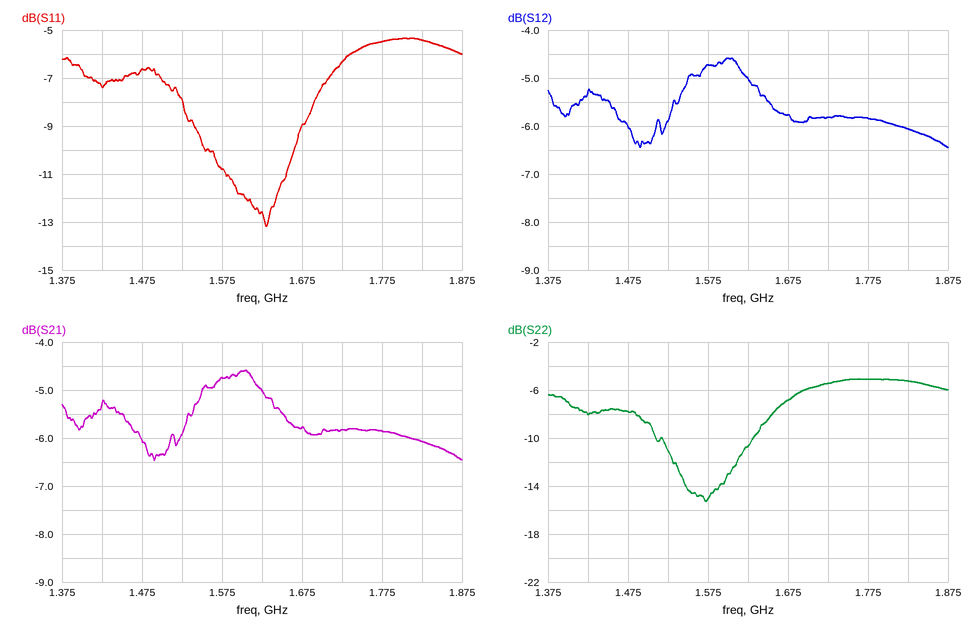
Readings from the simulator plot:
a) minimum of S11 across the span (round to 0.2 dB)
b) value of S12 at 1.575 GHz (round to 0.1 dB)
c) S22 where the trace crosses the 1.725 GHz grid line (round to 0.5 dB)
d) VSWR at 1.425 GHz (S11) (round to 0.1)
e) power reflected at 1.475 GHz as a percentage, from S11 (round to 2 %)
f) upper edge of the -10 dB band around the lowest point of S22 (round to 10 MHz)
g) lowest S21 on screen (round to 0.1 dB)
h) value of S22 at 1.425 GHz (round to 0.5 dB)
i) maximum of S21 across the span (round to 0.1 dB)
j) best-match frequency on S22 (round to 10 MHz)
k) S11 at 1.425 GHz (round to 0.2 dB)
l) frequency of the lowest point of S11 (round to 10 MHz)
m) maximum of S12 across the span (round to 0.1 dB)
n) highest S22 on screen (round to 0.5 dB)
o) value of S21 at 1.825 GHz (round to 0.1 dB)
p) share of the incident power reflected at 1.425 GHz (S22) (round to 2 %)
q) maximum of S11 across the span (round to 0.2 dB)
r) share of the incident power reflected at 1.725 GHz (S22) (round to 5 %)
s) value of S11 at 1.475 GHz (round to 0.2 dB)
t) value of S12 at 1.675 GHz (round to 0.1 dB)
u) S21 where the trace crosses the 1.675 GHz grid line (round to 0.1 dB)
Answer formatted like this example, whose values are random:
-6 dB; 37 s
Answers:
-13.2 dB; -4.7 dB; -5.5 dB; 2.5; 22 %; 1.63 GHz; -6.5 dB; -8.0 dB; -4.6 dB; 1.57 GHz; -7.4 dB; 1.63 GHz; -4.6 dB; -5.0 dB; -6.1 dB; 16 %; -5.4 dB; 30 %; -6.6 dB; -5.8 dB; -5.8 dB
